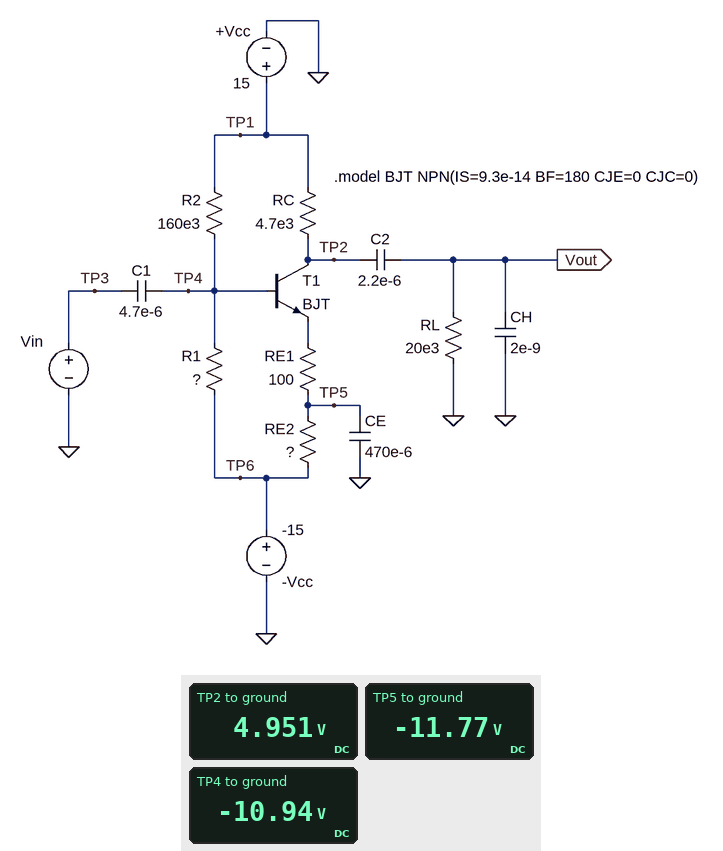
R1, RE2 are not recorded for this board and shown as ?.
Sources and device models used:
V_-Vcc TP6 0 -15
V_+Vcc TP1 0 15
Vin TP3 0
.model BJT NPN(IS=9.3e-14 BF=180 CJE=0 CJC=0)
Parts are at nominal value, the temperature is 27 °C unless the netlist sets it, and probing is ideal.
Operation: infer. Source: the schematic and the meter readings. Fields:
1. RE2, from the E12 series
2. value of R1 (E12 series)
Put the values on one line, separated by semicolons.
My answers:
1.5 kΩ; 27 kΩ
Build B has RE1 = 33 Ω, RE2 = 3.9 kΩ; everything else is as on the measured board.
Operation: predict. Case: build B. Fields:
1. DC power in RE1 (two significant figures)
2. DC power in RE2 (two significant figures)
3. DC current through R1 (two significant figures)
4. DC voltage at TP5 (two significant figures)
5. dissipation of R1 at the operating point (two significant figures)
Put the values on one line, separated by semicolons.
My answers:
28 µW; 3.3 mW; 160 µA; -11 V; 660 µW
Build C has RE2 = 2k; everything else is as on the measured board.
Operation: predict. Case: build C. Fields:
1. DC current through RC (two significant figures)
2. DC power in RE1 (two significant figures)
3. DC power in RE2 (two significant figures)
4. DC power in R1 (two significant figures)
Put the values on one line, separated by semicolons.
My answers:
1.7 mA; 280 µW; 5.6 mW; 630 µW
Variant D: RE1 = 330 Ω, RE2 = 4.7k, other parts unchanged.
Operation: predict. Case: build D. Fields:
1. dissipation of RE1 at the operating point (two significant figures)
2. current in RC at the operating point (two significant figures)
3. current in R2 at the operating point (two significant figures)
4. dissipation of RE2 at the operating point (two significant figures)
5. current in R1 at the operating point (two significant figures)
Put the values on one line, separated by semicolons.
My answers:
170 µW; 720 µA; 160 µA; 2.5 mW; 160 µA
